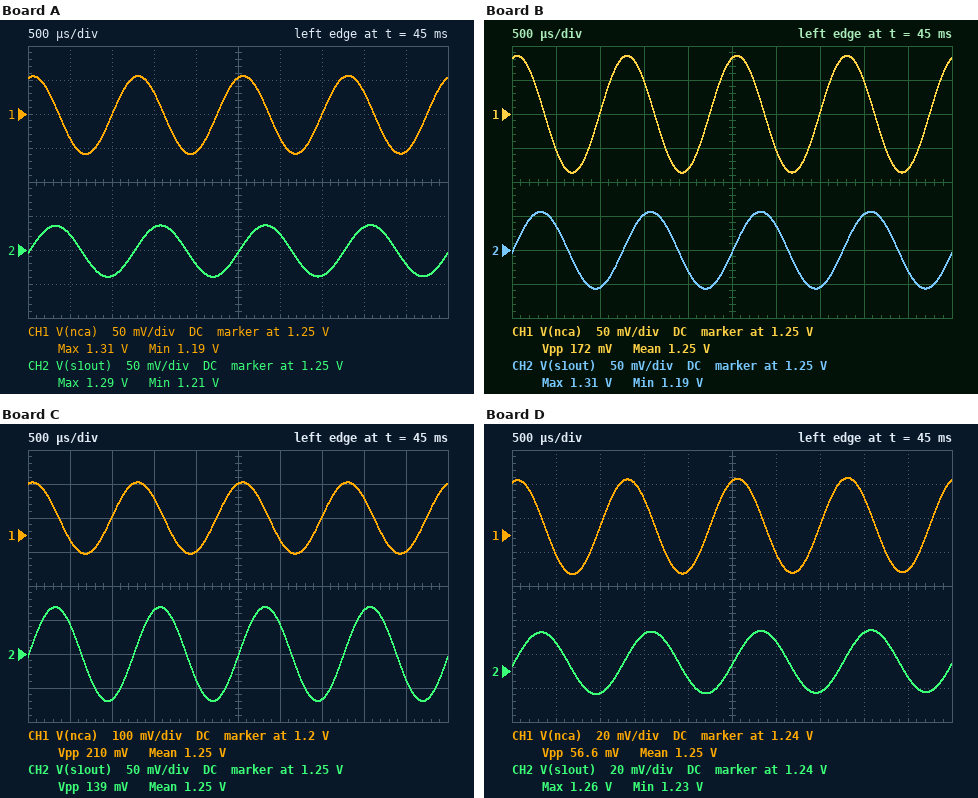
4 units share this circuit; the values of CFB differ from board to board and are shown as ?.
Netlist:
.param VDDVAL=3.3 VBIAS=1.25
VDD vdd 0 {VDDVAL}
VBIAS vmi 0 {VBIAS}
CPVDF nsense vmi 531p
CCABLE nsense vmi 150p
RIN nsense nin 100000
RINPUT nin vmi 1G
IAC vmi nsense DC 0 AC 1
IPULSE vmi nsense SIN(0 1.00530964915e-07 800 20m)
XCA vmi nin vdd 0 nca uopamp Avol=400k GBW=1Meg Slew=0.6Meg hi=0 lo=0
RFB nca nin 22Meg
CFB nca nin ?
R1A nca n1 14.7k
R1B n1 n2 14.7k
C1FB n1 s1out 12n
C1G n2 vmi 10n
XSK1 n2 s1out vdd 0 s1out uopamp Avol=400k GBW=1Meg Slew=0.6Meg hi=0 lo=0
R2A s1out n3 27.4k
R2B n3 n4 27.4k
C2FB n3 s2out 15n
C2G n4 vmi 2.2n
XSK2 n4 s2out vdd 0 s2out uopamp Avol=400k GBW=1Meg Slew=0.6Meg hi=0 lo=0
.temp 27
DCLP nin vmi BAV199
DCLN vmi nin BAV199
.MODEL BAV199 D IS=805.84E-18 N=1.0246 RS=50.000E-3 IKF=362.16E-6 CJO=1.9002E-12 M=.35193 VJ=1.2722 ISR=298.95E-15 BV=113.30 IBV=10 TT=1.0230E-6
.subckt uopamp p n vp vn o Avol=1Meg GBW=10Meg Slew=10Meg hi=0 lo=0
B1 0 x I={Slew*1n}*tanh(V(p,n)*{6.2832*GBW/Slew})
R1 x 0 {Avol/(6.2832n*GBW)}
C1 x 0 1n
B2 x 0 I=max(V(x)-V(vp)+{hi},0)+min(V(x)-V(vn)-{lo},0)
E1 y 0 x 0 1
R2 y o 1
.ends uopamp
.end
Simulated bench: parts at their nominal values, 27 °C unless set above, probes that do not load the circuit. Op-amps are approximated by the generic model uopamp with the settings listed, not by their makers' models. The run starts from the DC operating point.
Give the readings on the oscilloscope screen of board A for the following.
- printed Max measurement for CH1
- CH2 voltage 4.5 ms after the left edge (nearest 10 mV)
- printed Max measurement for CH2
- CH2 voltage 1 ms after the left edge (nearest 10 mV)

1.31 V
1.23 V
1.29 V
1.21 V
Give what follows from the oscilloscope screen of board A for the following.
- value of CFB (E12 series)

330 pF
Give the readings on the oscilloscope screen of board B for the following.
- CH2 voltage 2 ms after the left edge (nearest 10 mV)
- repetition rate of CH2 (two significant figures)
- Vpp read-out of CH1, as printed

1.22 V
800 Hz
172 mV
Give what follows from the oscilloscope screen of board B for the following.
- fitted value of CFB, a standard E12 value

220 pF
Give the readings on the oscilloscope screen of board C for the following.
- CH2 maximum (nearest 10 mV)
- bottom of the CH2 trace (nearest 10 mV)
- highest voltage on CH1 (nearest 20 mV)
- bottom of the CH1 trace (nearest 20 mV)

1.32 V
1.18 V
1.36 V
1.14 V
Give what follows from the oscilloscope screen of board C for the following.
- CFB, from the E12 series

180 pF
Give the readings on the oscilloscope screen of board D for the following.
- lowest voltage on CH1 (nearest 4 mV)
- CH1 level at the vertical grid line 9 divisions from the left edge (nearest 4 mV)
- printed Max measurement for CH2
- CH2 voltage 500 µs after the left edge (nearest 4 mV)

1.216 V
1.220 V
1.26 V
1.256 V
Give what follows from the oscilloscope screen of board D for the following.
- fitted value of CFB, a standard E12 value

680 pF
